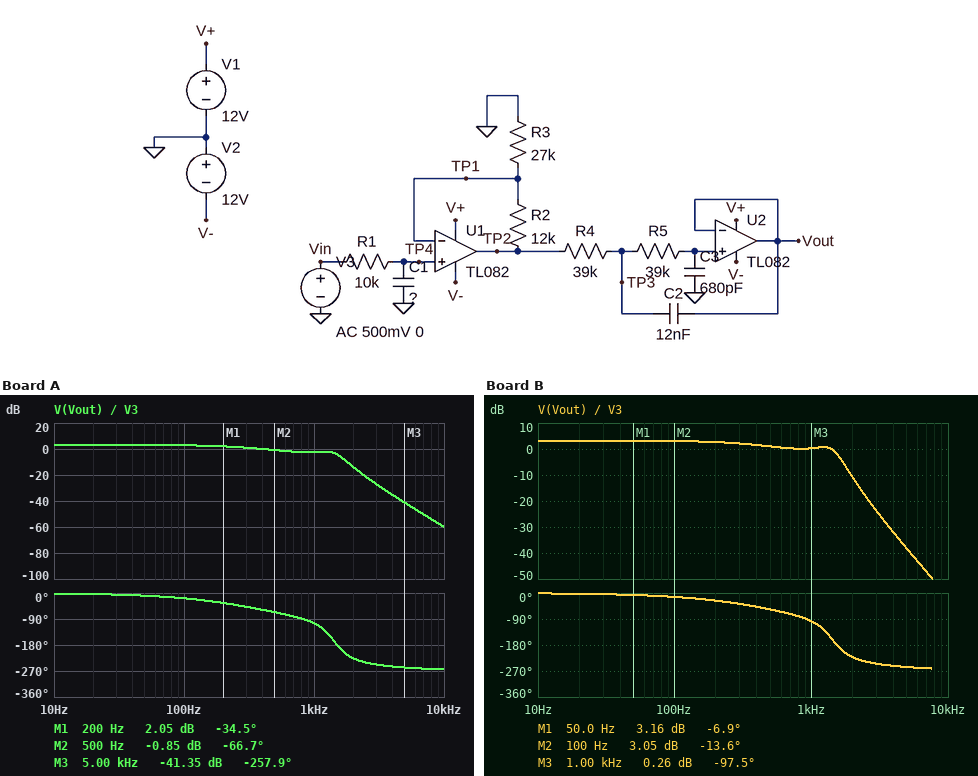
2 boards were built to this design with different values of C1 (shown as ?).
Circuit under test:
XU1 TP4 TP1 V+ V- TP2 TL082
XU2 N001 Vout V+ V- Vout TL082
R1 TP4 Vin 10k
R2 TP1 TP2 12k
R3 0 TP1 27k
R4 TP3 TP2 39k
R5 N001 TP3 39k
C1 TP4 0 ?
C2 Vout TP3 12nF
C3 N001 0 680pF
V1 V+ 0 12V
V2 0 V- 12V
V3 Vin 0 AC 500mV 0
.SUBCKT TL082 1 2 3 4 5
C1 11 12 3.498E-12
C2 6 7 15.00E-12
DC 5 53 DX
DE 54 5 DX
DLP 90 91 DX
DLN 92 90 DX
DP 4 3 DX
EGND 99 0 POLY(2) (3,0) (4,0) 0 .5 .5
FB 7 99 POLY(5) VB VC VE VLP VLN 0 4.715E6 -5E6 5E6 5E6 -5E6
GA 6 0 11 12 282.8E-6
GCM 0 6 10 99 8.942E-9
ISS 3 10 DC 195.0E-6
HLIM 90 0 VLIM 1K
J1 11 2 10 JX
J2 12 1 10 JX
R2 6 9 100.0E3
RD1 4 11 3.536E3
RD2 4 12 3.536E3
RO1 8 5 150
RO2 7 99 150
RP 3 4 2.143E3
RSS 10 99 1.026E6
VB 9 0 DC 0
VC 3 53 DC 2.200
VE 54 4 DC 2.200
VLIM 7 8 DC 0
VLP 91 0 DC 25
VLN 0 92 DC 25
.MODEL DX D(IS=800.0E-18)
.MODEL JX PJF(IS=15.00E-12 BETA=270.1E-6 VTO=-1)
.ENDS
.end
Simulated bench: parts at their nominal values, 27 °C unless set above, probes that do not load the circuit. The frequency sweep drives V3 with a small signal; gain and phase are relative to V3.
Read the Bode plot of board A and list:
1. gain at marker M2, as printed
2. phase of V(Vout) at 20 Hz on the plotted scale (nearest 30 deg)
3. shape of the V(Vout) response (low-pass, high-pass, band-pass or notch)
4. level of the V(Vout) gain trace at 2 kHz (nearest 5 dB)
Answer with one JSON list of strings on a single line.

["-0.85 dB", "0 deg", "low-pass", "-15 dB"]
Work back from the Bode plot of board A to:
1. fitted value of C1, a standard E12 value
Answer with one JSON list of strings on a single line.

["47 nF"]
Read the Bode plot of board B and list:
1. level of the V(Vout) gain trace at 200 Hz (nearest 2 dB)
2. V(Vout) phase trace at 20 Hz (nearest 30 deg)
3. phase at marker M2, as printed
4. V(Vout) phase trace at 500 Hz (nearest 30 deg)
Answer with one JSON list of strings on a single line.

["2 dB", "0 deg", "-13.6 deg", "-60 deg"]
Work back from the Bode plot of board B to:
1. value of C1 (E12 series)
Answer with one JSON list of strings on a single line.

["33 nF"]
